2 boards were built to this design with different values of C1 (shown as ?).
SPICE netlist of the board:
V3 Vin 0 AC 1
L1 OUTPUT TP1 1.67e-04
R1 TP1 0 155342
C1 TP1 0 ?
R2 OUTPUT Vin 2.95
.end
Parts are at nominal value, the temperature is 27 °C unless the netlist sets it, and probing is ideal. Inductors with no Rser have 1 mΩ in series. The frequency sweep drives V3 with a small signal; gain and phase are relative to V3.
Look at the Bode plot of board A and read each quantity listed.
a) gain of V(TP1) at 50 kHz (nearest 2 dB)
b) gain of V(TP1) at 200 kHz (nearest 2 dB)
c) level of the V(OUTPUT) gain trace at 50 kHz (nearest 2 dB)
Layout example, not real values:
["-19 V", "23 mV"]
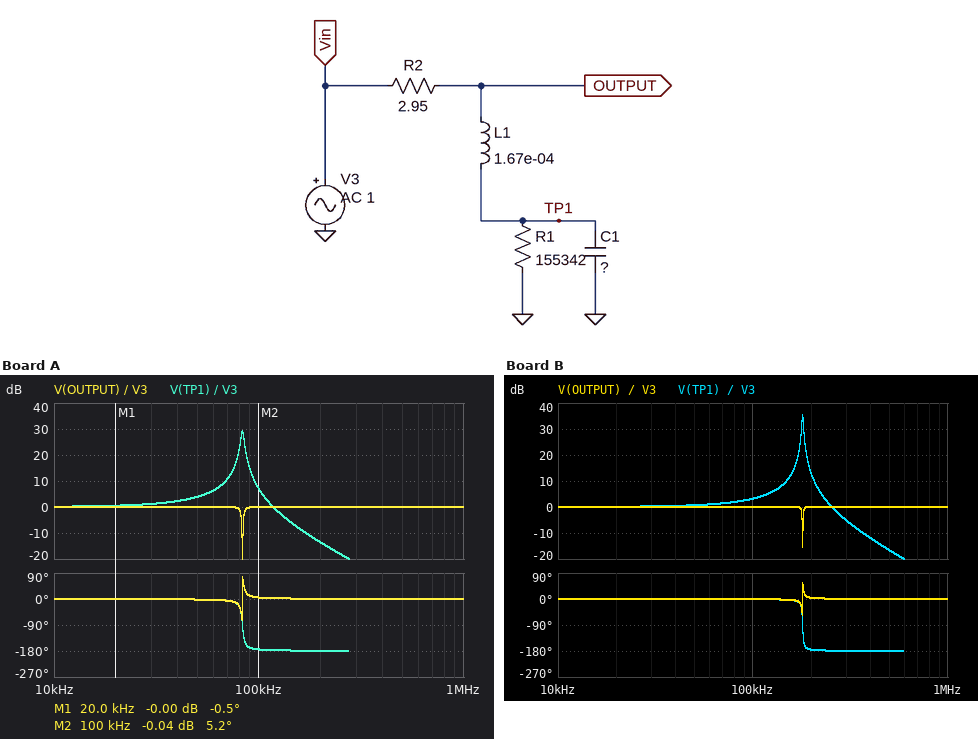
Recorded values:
["4 dB", "-14 dB", "0 dB"]
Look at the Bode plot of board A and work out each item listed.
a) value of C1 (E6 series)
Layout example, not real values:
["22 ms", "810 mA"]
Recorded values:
["22 nF"]
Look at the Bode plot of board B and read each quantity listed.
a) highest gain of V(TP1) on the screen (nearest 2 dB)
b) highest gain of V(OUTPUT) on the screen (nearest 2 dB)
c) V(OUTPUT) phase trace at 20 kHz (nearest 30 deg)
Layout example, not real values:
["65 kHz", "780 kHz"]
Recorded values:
["36 dB", "0 dB", "0 deg"]
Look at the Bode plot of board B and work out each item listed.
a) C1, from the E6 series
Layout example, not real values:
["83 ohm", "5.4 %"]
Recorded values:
["4.7 nF"]
